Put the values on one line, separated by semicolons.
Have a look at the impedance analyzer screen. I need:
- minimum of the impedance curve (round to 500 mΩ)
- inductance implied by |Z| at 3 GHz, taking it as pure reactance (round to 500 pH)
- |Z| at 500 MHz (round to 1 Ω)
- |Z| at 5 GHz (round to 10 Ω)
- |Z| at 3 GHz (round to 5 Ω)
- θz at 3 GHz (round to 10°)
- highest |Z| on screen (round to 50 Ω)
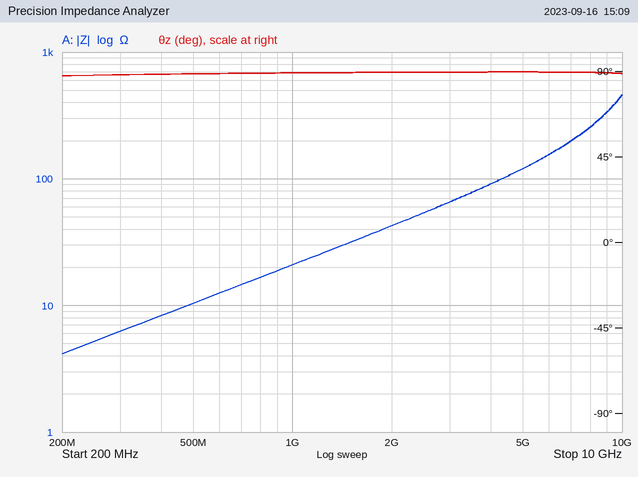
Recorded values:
4.0 Ω; 3.5 nH; 10 Ω; 120 Ω; 65 Ω; 90°; 450 Ω
